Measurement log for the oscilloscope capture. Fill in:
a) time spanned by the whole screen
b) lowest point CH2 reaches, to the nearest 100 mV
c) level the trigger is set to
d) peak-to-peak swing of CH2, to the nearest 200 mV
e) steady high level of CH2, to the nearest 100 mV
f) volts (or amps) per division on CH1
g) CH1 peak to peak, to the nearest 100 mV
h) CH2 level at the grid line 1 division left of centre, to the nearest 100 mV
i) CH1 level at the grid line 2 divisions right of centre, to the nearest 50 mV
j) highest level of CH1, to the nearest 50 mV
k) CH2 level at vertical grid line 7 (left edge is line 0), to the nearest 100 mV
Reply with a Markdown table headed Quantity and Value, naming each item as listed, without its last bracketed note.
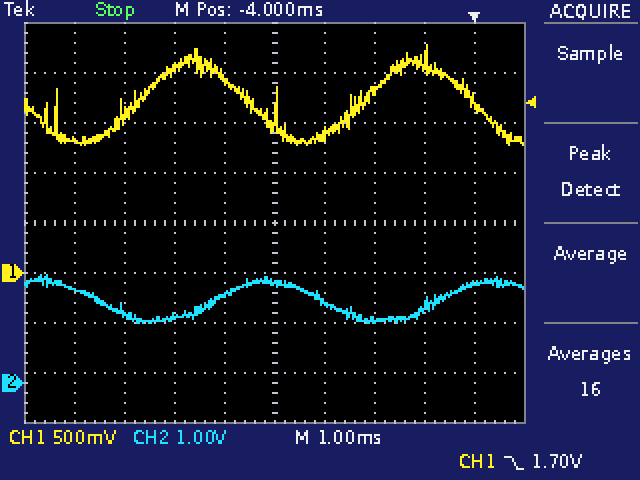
| Quantity | Value |
|---|---|
| time spanned by the whole screen | 10 ms |
| lowest point CH2 reaches, to the nearest 100 mV | 1.2 V |
| level the trigger is set to | 1.70 V |
| peak-to-peak swing of CH2, to the nearest 200 mV | 1.0 V |
| steady high level of CH2, to the nearest 100 mV | 2.0 V |
| volts (or amps) per division on CH1 | 500 mV |
| CH1 peak to peak, to the nearest 100 mV | 1.00 V |
| CH2 level at the grid line 1 division left of centre, to the nearest 100 mV | 1.8 V |
| CH1 level at the grid line 2 divisions right of centre, to the nearest 50 mV | 1.80 V |
| highest level of CH1, to the nearest 50 mV | 2.30 V |
| CH2 level at vertical grid line 7 (left edge is line 0), to the nearest 100 mV | 1.3 V |
